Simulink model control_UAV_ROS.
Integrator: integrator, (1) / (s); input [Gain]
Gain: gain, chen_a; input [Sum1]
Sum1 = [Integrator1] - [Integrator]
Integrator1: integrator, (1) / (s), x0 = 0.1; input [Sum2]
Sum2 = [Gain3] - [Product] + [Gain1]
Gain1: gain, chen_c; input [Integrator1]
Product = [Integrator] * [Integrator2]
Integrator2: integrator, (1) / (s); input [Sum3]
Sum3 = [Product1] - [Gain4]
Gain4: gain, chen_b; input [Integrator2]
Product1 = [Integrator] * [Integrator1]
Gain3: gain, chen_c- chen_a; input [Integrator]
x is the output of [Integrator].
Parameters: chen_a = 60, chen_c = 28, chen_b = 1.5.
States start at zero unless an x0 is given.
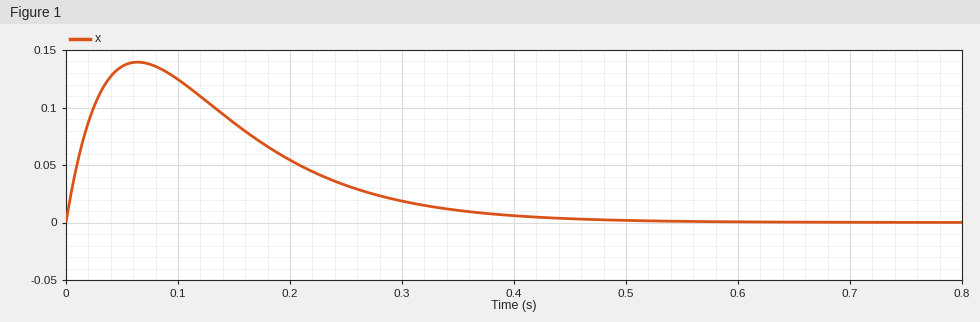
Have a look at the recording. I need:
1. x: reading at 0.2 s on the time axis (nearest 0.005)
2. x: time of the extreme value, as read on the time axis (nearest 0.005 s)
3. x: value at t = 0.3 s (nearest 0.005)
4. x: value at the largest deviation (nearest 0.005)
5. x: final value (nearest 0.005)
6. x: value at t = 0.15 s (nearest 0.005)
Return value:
0.055
0.065 s
0.020
0.140
0.000
0.085
